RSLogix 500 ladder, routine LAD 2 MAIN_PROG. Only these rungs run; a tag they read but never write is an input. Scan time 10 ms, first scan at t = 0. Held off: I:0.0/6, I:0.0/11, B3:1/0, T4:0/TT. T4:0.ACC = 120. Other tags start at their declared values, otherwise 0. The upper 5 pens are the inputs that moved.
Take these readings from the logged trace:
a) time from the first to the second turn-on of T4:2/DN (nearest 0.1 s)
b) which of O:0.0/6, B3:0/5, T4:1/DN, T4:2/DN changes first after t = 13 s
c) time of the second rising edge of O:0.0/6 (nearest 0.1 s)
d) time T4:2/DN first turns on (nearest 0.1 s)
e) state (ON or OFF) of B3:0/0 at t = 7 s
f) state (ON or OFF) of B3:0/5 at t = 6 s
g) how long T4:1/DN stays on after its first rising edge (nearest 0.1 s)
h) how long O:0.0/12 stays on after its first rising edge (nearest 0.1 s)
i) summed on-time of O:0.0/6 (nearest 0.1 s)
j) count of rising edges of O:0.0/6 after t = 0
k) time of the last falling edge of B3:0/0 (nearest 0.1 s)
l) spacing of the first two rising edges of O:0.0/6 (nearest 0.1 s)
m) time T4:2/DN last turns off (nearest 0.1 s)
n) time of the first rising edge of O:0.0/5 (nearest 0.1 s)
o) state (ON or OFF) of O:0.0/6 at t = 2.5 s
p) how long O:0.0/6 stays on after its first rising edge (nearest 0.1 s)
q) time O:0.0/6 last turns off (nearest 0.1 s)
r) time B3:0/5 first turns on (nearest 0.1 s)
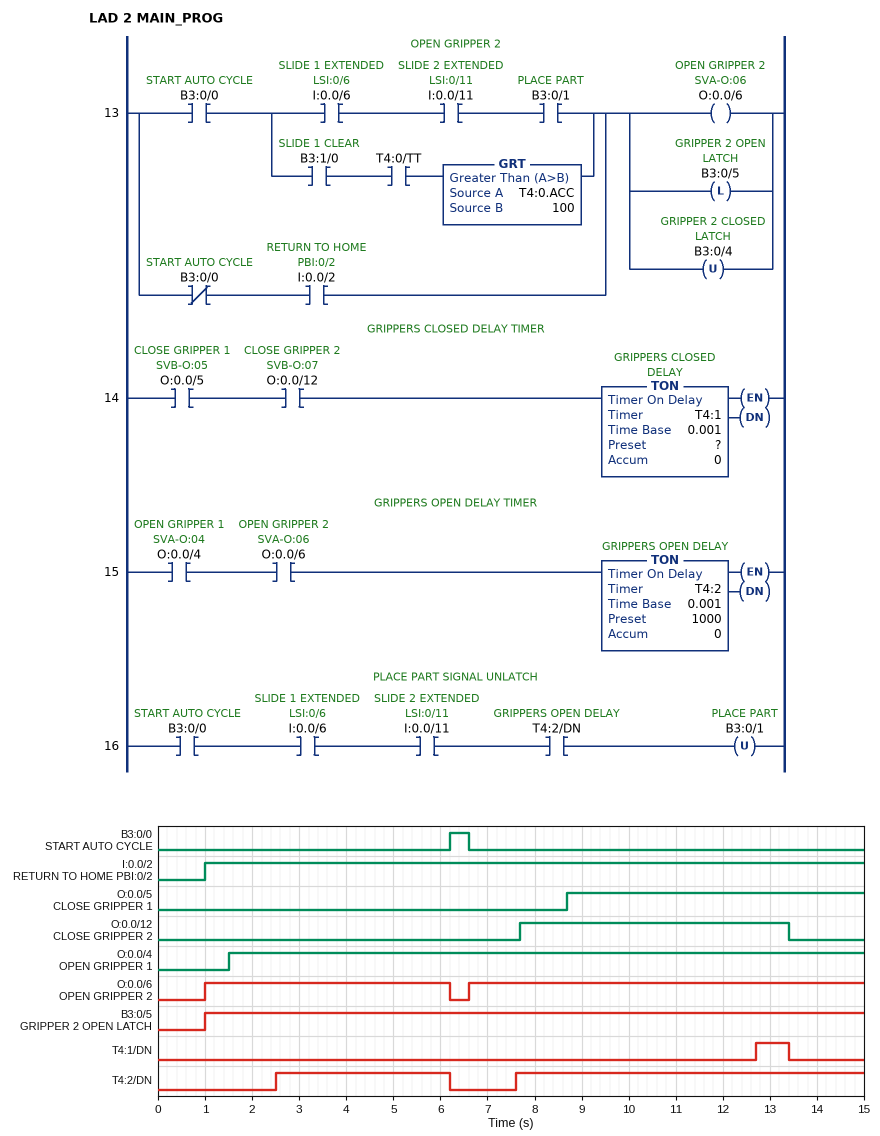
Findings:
5.1 s
T4:1/DN
6.6 s
2.5 s
OFF
ON
0.7 s
5.7 s
13.6 s
2
6.6 s
5.6 s
6.2 s
8.7 s
ON
5.2 s
6.2 s
1.0 s
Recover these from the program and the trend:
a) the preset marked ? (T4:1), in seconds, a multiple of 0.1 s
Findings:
4.0 s
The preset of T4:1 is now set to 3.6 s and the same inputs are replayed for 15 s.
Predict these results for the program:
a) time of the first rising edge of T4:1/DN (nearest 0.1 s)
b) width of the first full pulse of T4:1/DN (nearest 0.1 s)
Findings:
12.3 s
1.1 s
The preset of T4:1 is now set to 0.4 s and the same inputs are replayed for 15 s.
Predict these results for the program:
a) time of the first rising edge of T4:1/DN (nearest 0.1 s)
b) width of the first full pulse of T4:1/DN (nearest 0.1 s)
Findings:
9.1 s
4.3 s
